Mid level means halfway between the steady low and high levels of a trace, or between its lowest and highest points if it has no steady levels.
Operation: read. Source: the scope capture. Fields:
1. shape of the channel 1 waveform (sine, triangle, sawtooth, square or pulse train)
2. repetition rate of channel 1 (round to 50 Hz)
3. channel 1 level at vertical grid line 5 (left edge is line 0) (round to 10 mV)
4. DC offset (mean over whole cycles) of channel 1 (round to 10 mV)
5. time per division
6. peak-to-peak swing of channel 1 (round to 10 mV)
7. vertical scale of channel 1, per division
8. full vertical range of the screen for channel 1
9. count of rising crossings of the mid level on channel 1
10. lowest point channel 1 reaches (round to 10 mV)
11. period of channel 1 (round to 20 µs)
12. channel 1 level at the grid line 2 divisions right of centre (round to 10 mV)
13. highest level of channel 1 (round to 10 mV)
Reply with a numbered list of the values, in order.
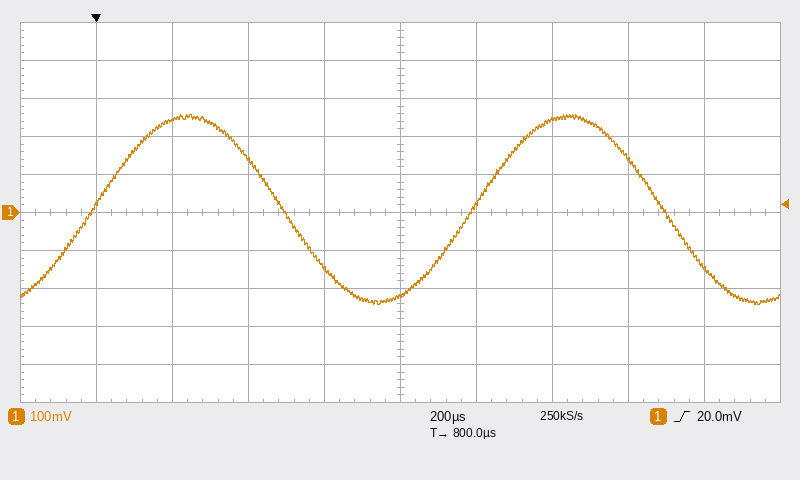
1. sine
2. 1.00 kHz
3. -220 mV
4. 10 mV
5. 200 µs
6. 500 mV
7. 100 mV
8. 1 V
9. 2
10. -240 mV
11. 1.00 ms
12. 240 mV
13. 260 mV
